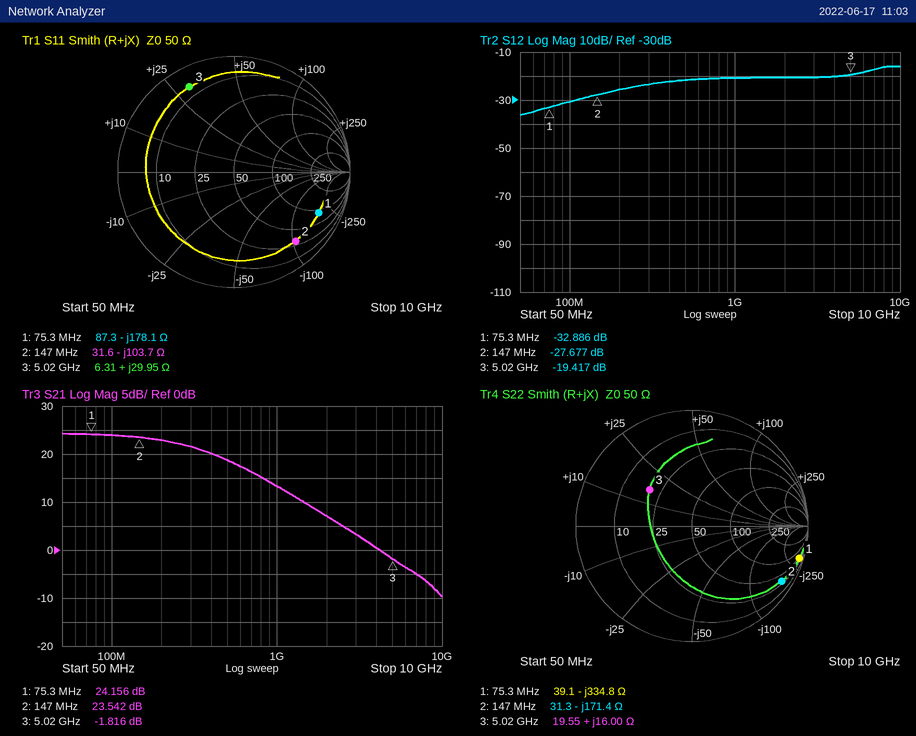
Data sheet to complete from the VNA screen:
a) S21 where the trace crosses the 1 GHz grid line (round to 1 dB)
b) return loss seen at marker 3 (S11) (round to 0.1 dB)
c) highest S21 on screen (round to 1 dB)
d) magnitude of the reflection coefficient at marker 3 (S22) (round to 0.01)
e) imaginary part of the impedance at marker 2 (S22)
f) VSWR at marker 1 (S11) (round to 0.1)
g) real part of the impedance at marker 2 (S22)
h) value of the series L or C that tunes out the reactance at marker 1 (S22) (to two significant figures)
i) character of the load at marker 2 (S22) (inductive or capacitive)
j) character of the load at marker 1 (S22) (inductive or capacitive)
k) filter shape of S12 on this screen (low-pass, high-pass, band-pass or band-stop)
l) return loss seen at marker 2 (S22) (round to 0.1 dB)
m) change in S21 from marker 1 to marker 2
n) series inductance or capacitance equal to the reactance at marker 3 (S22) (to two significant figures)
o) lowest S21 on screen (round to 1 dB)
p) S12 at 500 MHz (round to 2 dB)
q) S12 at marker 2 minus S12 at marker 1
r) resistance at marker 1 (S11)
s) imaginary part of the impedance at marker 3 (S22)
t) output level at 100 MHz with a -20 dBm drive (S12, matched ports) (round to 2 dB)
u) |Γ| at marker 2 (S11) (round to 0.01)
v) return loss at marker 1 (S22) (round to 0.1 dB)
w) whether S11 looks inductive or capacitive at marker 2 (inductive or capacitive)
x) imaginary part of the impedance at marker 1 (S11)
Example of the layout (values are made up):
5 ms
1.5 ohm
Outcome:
13 dB
1.6 dB
24 dB
0.48
-171.4 Ω
9.5
31.3 Ω
710 nH
capacitive
capacitive
high-pass
0.8 dB
-0.614 dB
510 pH
-10 dB
-22 dB
5.209 dB
87.3 Ω
+16.00 Ω
-50 dBm
0.80
0.3 dB
capacitive
-178.1 Ω
